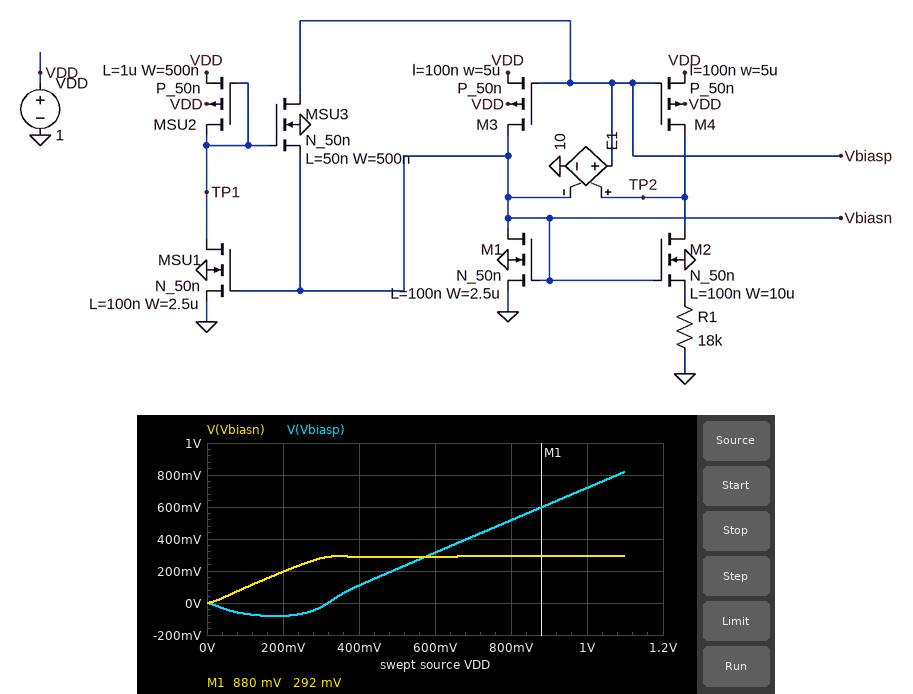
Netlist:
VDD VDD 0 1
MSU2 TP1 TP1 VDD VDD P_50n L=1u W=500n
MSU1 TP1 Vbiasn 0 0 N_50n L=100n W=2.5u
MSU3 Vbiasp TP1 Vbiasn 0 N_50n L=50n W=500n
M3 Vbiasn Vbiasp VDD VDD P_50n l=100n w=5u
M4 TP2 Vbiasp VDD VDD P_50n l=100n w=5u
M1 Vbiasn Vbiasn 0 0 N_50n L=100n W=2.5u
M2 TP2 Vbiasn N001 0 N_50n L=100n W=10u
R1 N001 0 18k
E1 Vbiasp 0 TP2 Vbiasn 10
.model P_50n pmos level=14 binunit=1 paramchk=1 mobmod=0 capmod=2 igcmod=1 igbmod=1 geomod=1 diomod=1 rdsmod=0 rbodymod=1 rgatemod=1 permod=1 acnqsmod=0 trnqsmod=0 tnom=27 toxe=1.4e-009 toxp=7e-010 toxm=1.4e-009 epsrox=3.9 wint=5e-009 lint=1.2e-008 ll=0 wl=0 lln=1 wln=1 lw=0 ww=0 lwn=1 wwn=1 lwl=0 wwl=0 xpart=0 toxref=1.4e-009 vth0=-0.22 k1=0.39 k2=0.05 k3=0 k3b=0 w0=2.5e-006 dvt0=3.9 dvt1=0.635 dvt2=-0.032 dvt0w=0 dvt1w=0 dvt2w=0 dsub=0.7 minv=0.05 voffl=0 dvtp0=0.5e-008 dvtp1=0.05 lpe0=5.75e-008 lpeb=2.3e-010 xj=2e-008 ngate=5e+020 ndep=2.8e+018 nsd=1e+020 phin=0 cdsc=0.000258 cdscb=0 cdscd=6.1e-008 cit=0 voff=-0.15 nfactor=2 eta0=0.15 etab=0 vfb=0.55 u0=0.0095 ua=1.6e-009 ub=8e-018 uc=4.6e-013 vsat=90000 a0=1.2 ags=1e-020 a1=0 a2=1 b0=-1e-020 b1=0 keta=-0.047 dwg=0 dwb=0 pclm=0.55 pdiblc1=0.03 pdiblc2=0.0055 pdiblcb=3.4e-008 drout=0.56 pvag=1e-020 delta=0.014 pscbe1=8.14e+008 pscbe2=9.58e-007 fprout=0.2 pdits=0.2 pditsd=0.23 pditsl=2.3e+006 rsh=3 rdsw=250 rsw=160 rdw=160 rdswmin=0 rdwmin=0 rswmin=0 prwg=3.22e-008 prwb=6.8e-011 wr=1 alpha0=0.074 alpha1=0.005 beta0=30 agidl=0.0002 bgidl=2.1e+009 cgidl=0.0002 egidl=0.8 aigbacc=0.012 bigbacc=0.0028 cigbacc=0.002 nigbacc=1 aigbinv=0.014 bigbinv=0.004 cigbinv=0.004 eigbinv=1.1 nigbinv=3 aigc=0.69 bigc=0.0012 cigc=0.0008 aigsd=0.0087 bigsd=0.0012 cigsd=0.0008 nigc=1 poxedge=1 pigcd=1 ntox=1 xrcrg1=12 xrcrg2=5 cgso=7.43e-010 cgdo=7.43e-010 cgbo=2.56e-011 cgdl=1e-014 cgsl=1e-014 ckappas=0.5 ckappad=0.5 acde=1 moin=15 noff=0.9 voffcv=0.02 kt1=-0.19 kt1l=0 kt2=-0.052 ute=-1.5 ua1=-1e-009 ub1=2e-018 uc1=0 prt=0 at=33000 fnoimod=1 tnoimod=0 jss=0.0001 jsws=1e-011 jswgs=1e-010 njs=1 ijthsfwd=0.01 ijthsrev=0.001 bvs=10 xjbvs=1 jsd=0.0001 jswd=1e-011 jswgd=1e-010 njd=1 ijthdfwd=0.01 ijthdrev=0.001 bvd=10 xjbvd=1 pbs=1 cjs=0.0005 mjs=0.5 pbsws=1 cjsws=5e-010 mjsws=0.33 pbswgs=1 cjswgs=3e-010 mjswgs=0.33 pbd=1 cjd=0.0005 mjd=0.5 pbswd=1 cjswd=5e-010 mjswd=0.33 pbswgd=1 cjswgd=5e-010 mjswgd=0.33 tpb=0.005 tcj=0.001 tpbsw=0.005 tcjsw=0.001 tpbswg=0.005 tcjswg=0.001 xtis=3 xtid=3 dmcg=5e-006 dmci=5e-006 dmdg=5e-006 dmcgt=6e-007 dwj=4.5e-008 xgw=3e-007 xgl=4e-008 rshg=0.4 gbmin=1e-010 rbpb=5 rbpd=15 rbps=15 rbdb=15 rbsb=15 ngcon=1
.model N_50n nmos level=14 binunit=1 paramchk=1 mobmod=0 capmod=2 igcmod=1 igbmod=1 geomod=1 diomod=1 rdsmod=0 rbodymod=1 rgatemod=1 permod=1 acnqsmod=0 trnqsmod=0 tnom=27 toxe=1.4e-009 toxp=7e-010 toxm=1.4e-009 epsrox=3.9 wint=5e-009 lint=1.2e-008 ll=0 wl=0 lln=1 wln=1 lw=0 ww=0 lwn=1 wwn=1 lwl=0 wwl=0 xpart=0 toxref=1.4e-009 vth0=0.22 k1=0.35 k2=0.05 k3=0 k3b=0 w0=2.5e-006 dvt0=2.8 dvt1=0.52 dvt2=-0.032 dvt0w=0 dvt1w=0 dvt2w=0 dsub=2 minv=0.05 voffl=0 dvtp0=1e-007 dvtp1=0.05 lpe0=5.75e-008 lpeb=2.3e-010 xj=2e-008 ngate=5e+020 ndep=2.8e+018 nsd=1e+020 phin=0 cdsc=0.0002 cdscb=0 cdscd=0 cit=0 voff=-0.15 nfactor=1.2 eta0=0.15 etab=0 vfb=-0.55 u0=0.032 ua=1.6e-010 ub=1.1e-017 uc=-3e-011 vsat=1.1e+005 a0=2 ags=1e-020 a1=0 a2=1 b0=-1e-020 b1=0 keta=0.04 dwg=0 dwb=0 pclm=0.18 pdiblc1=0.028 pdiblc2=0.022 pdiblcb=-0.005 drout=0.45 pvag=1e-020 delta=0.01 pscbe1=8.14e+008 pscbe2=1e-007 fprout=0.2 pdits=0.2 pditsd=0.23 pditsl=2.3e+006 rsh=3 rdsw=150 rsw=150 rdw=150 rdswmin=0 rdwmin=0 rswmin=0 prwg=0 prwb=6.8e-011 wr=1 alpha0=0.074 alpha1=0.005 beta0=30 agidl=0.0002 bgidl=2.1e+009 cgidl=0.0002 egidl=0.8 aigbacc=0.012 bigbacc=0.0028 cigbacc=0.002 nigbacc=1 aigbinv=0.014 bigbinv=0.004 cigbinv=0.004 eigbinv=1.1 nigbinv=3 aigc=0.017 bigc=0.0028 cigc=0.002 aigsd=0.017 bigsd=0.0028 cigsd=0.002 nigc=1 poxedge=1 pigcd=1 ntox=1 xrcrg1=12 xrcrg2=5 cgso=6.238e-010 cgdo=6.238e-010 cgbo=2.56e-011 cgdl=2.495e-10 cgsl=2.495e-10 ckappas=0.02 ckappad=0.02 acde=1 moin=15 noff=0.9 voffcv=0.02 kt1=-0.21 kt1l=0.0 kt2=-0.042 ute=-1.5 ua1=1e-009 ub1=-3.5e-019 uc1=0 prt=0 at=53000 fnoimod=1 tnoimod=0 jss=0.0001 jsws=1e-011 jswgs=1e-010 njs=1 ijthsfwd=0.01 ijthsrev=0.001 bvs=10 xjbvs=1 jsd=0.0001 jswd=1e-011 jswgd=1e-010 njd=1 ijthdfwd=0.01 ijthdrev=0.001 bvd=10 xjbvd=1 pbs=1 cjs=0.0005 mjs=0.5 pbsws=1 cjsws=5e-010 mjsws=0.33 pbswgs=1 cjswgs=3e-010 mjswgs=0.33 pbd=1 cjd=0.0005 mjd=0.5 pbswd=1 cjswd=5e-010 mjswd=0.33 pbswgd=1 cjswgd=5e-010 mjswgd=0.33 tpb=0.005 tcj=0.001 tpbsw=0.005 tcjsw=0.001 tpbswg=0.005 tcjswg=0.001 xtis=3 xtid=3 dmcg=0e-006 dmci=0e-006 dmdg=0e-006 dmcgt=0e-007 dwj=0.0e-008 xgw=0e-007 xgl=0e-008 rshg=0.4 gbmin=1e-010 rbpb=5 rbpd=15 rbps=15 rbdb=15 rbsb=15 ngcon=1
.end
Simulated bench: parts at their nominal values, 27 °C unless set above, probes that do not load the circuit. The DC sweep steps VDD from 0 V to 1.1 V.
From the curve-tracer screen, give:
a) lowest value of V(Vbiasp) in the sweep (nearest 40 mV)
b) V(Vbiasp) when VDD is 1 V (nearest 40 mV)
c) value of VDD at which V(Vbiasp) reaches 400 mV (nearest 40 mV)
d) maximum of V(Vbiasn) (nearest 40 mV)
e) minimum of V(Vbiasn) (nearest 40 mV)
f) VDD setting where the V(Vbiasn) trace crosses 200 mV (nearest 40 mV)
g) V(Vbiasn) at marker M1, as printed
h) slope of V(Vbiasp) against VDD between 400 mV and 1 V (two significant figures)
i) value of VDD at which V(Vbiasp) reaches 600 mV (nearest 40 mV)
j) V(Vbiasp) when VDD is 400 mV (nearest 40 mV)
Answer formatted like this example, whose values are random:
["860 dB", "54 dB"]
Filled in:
["-80 mV", "720 mV", "680 mV", "280 mV", "0 V", "200 mV", "292 mV", "1.0 V/V", "880 mV", "120 mV"]
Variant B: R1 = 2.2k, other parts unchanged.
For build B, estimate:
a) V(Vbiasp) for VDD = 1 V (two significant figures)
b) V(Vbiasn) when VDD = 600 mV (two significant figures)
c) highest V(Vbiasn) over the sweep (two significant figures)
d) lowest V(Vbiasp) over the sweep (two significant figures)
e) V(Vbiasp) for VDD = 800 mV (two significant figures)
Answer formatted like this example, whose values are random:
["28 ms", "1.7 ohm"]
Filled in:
["570 mV", "420 mV", "430 mV", "-130 mV", "370 mV"]
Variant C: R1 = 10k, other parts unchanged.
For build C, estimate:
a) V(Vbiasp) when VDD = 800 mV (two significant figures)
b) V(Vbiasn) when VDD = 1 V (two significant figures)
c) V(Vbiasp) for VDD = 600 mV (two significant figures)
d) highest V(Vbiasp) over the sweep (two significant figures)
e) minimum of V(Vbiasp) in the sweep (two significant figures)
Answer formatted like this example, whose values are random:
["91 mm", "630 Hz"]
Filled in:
["480 mV", "320 mV", "280 mV", "790 mV", "-90 mV"]
